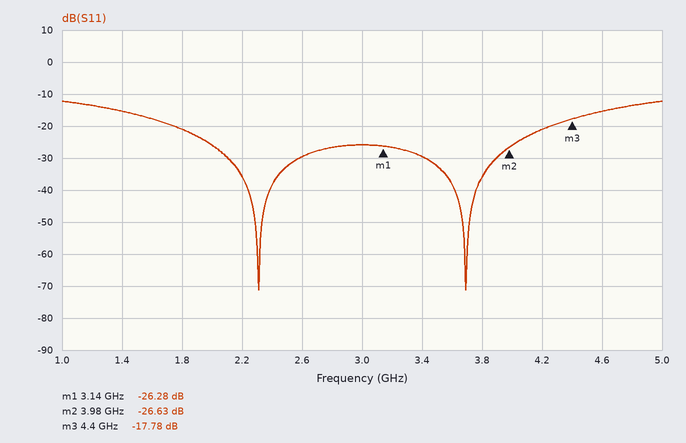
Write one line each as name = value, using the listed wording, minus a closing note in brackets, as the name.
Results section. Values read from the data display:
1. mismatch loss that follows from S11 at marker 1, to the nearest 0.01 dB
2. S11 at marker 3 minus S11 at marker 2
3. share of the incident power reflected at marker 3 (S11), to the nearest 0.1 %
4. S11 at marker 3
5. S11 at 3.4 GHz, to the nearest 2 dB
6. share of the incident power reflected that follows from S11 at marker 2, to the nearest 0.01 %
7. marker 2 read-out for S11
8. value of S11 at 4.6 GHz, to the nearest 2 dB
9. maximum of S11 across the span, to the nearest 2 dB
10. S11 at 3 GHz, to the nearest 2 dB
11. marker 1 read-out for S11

mismatch loss that follows from S11 at marker 1, to the nearest 0.01 dB = 0.01 dB
S11 at marker 3 minus S11 at marker 2 = 8.85 dB
share of the incident power reflected at marker 3 (S11), to the nearest 0.1 % = 1.7 %
S11 at marker 3 = -17.78 dB
S11 at 3.4 GHz, to the nearest 2 dB = -30 dB
share of the incident power reflected that follows from S11 at marker 2, to the nearest 0.01 % = 0.22 %
marker 2 read-out for S11 = -26.63 dB
value of S11 at 4.6 GHz, to the nearest 2 dB = -16 dB
maximum of S11 across the span, to the nearest 2 dB = -12 dB
S11 at 3 GHz, to the nearest 2 dB = -26 dB
marker 1 read-out for S11 = -26.28 dB
